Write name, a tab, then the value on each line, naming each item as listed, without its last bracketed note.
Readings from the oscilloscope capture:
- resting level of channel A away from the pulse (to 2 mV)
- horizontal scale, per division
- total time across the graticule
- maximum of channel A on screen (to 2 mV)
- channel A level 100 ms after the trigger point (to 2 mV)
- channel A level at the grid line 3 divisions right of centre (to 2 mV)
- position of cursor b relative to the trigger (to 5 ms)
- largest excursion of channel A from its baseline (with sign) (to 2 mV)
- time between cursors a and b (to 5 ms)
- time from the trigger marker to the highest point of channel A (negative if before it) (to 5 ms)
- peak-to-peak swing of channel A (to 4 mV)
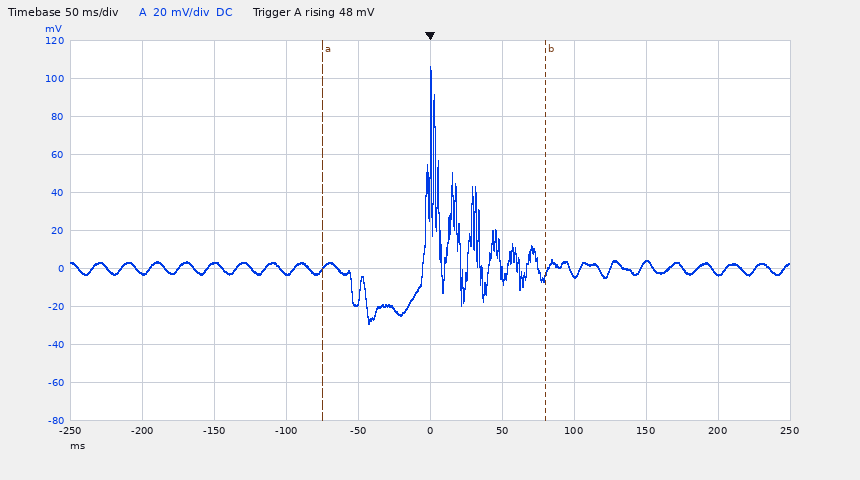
resting level of channel A away from the pulse	0 mV
horizontal scale, per division	50 ms
total time across the graticule	500 ms
maximum of channel A on screen	106 mV
channel A level 100 ms after the trigger point	-4 mV
channel A level at the grid line 3 divisions right of centre	4 mV
position of cursor b relative to the trigger	+80 ms
largest excursion of channel A from its baseline (with sign)	+106 mV
time between cursors a and b	155 ms
time from the trigger marker to the highest point of channel A (negative if before it)	0 ms
peak-to-peak swing of channel A	136 mV
